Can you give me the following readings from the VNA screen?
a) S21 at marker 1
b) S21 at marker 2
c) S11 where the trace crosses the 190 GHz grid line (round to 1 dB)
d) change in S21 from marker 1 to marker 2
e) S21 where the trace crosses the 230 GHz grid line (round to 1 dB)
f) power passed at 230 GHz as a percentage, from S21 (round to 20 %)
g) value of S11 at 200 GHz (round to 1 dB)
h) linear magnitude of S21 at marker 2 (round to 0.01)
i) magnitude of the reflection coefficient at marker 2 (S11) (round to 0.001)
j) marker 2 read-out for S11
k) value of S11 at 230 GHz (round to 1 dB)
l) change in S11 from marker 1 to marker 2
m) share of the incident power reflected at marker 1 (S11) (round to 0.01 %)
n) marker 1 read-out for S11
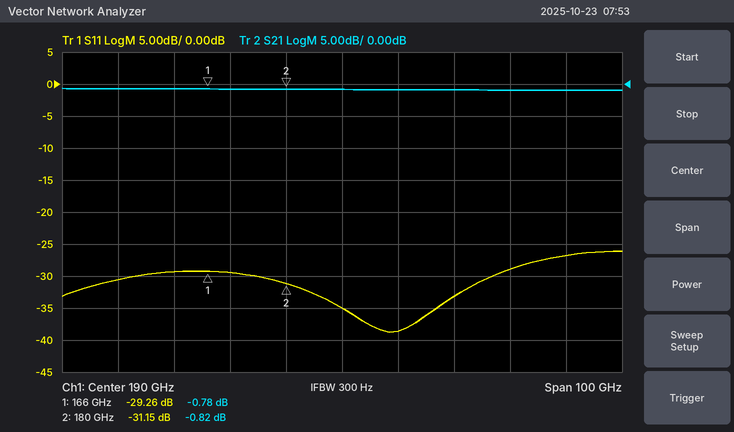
-0.78 dB
-0.82 dB
-35 dB
-0.04 dB
-1 dB
80 %
-39 dB
0.91
0.028
-31.15 dB
-27 dB
-1.89 dB
0.12 %
-29.26 dB
